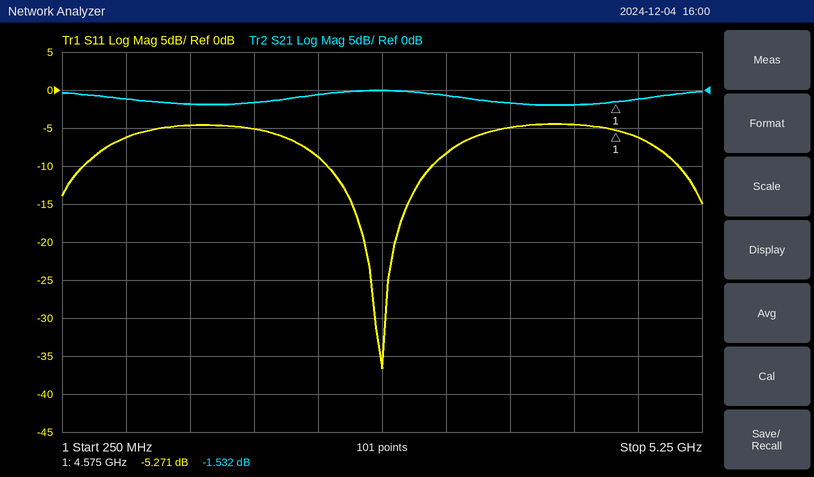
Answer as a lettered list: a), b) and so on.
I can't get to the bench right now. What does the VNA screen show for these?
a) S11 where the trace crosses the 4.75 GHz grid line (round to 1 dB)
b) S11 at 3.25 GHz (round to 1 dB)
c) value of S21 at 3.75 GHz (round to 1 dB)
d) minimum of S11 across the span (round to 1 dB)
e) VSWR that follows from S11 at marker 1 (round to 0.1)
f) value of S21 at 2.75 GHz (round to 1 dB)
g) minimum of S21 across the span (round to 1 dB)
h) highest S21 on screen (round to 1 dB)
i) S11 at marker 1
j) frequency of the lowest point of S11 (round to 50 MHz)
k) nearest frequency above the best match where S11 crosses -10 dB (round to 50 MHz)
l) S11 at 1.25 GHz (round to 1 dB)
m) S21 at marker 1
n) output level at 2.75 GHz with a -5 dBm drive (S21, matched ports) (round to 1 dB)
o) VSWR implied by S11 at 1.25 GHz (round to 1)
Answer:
a) -6 dB
b) -8 dB
c) -2 dB
d) -37 dB
e) 3.4
f) 0 dB
g) -2 dB
h) 0 dB
i) -5.271 dB
j) 2.75 GHz
k) 3.15 GHz
l) -5 dB
m) -1.532 dB
n) -5 dBm
o) 4
